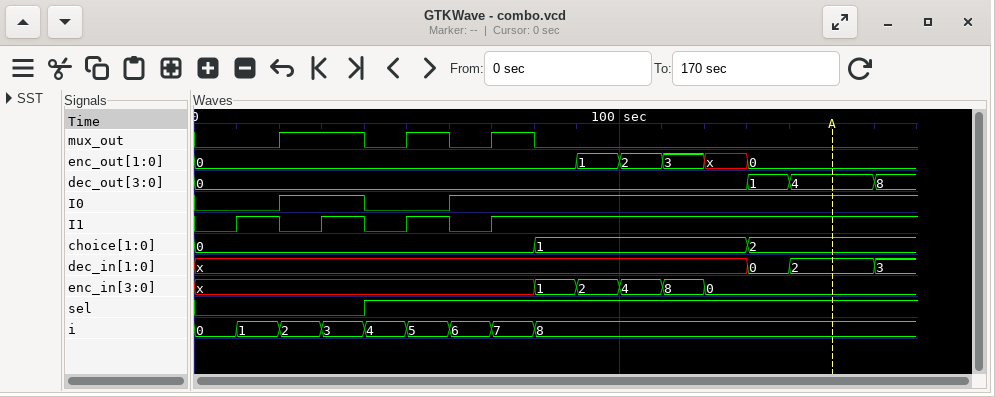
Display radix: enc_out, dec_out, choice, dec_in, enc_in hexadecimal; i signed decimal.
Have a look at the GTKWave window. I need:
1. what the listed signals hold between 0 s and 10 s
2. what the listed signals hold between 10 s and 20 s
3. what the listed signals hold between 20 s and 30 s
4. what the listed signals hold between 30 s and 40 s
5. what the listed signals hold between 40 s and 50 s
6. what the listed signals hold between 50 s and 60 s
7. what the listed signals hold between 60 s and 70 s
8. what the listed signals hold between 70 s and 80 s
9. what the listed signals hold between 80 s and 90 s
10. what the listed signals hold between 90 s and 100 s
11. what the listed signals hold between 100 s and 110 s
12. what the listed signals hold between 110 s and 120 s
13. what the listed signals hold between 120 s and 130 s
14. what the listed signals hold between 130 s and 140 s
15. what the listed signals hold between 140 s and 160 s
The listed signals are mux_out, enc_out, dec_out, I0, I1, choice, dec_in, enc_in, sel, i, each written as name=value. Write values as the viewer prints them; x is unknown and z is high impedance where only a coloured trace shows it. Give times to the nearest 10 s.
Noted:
mux_out=0, enc_out=0, dec_out=0, I0=0, I1=0, choice=0, dec_in=x, enc_in=x, sel=0, i=0
mux_out=0, enc_out=0, dec_out=0, I0=0, I1=1, choice=0, dec_in=x, enc_in=x, sel=0, i=1
mux_out=1, enc_out=0, dec_out=0, I0=1, I1=0, choice=0, dec_in=x, enc_in=x, sel=0, i=2
mux_out=1, enc_out=0, dec_out=0, I0=1, I1=1, choice=0, dec_in=x, enc_in=x, sel=0, i=3
mux_out=0, enc_out=0, dec_out=0, I0=0, I1=0, choice=0, dec_in=x, enc_in=x, sel=1, i=4
mux_out=1, enc_out=0, dec_out=0, I0=0, I1=1, choice=0, dec_in=x, enc_in=x, sel=1, i=5
mux_out=0, enc_out=0, dec_out=0, I0=1, I1=0, choice=0, dec_in=x, enc_in=x, sel=1, i=6
mux_out=1, enc_out=0, dec_out=0, I0=1, I1=1, choice=0, dec_in=x, enc_in=x, sel=1, i=7
mux_out=0, enc_out=0, dec_out=0, I0=1, I1=1, choice=1, dec_in=x, enc_in=1, sel=1, i=8
mux_out=0, enc_out=1, dec_out=0, I0=1, I1=1, choice=1, dec_in=x, enc_in=2, sel=1, i=8
mux_out=0, enc_out=2, dec_out=0, I0=1, I1=1, choice=1, dec_in=x, enc_in=4, sel=1, i=8
mux_out=0, enc_out=3, dec_out=0, I0=1, I1=1, choice=1, dec_in=x, enc_in=8, sel=1, i=8
mux_out=0, enc_out=x, dec_out=0, I0=1, I1=1, choice=1, dec_in=x, enc_in=0, sel=1, i=8
mux_out=0, enc_out=0, dec_out=1, I0=1, I1=1, choice=2, dec_in=0, enc_in=0, sel=1, i=8
mux_out=0, enc_out=0, dec_out=4, I0=1, I1=1, choice=2, dec_in=2, enc_in=0, sel=1, i=8
